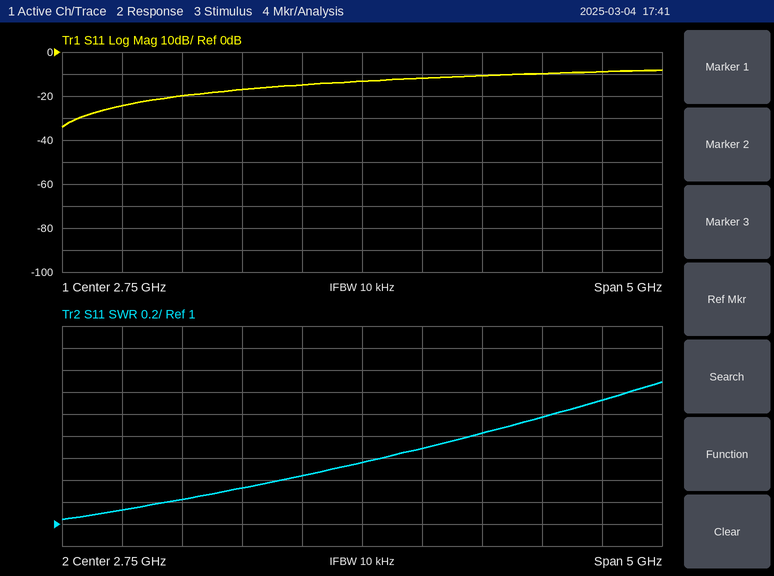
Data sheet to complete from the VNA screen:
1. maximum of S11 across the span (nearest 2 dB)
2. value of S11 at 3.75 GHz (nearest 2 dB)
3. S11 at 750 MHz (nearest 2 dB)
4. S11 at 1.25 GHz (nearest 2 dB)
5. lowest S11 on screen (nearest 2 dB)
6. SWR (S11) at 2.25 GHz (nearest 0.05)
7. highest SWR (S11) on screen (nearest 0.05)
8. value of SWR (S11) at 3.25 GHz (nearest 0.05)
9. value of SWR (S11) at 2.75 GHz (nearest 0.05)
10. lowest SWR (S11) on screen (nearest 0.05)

-8 dB
-10 dB
-24 dB
-20 dB
-34 dB
1.45
2.30
1.70
1.55
1.05
